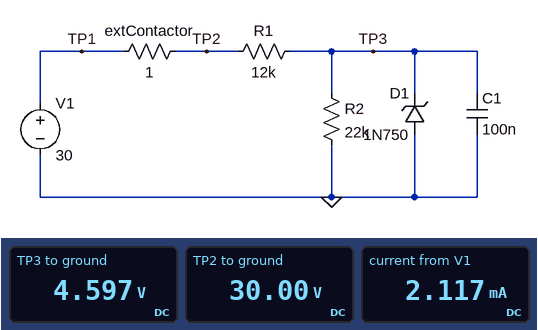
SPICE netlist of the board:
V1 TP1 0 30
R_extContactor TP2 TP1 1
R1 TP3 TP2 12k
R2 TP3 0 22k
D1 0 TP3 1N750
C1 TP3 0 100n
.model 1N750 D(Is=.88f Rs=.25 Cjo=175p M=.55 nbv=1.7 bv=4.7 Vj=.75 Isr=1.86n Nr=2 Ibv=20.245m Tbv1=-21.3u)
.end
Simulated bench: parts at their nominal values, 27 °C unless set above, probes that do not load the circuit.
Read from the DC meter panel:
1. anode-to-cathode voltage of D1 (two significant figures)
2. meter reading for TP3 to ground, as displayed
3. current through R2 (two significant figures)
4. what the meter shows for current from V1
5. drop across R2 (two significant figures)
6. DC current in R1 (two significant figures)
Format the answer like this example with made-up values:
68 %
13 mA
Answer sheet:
-4.6 V
4.597 V
210 µA
2.117 mA
4.6 V
2.1 mA
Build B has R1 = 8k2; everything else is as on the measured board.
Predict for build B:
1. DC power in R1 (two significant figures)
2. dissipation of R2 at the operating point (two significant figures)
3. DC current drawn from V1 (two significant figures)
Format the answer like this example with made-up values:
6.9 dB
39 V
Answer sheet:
79 mW
970 µW
3.1 mA
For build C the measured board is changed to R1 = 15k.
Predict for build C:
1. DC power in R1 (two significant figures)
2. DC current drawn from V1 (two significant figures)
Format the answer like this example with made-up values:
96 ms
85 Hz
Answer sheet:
43 mW
1.7 mA
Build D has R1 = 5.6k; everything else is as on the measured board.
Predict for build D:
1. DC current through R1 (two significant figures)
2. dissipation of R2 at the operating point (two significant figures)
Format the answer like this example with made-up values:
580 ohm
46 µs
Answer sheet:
4.5 mA
980 µW
